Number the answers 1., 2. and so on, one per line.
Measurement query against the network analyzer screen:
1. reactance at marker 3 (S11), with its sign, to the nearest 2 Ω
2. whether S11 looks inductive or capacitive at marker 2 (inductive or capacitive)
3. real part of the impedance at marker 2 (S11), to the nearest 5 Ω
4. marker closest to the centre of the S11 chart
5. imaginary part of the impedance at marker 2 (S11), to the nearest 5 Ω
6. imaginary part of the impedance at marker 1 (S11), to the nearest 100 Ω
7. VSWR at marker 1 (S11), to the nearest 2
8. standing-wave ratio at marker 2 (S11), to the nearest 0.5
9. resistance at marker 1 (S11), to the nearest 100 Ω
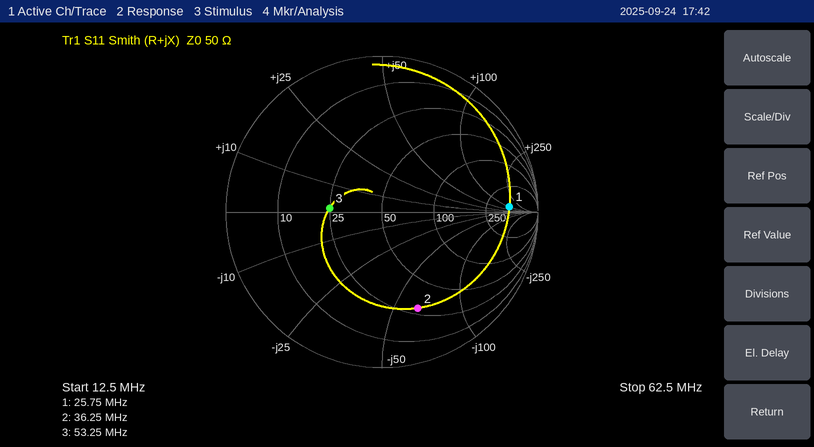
1. +2 Ω
2. capacitive
3. 30 Ω
4. marker 3
5. -65 Ω
6. +100 Ω
7. 10
8. 5.0
9. 500 Ω
